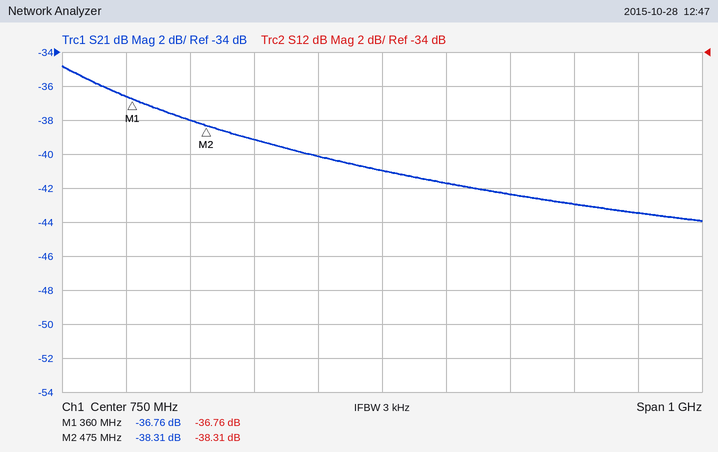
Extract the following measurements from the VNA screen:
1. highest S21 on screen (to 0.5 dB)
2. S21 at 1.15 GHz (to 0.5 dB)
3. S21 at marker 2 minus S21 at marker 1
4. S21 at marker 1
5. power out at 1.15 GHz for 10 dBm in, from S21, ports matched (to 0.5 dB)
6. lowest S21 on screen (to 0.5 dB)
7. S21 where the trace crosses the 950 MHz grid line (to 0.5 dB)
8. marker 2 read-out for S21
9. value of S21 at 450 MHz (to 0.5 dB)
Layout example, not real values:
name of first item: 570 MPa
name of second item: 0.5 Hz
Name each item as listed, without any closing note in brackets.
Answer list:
highest S21 on screen: -35.0 dB
S21 at 1.15 GHz: -43.5 dB
S21 at marker 2 minus S21 at marker 1: -1.55 dB
S21 at marker 1: -36.76 dB
power out at 1.15 GHz for 10 dBm in, from S21, ports matched: -33.5 dBm
lowest S21 on screen: -44.0 dB
S21 where the trace crosses the 950 MHz grid line: -42.5 dB
marker 2 read-out for S21: -38.31 dB
value of S21 at 450 MHz: -38.0 dB
